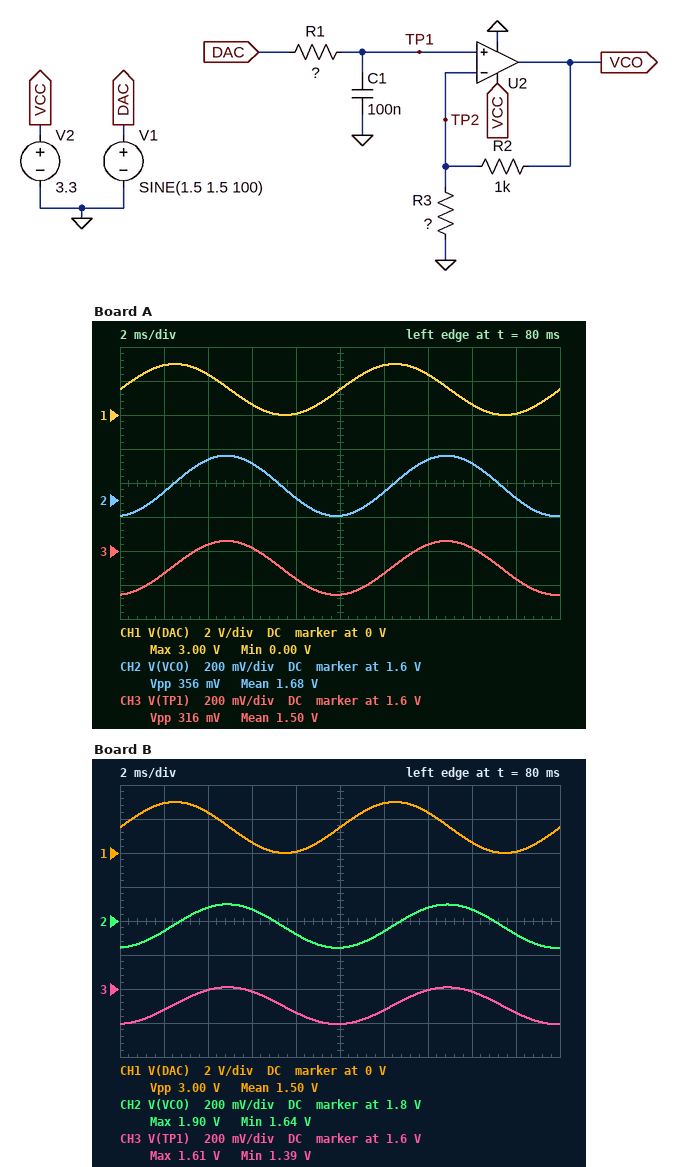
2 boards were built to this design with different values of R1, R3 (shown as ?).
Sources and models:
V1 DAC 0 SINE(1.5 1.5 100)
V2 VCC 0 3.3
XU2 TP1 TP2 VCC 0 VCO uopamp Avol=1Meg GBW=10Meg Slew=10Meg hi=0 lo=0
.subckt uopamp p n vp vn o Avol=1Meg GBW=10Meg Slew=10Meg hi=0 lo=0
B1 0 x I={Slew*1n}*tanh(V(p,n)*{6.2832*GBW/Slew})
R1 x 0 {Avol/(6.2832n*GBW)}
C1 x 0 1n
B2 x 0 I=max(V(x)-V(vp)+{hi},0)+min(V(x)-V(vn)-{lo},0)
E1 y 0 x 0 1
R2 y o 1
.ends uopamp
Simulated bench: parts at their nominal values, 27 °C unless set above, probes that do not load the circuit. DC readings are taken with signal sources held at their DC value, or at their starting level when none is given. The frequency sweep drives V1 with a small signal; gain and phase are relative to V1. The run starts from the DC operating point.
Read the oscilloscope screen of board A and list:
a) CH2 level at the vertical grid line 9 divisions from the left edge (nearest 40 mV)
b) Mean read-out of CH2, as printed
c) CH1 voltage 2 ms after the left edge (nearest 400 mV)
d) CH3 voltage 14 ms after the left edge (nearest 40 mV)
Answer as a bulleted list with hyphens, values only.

- 1.60 V
- 1.68 V
- 2.8 V
- 1.64 V
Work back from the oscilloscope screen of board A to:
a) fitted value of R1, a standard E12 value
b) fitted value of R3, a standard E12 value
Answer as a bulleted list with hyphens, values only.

- 150 kΩ
- 8.2 kΩ
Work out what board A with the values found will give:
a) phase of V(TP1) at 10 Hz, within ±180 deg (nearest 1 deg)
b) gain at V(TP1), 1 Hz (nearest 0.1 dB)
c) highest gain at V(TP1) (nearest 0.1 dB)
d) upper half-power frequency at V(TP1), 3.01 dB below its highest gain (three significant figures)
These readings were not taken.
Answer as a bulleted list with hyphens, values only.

- -43 deg
- 0 dB
- 0 dB
- 10.6 Hz
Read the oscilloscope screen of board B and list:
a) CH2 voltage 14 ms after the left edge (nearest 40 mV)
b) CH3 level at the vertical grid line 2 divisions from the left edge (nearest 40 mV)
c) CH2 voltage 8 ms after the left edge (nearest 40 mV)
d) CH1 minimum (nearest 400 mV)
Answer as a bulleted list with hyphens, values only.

- 1.88 V
- 1.60 V
- 1.72 V
- 0 V
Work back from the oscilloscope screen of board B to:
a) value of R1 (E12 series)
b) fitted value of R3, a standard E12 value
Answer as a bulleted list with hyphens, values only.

- 220 kΩ
- 5.6 kΩ
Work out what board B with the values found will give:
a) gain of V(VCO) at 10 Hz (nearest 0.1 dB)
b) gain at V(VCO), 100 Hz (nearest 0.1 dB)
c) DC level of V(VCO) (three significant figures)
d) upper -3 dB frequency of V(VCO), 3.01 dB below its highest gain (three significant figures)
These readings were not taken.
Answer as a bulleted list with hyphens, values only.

- -3.2 dB
- -21.4 dB
- 1.77 V
- 7.23 Hz
